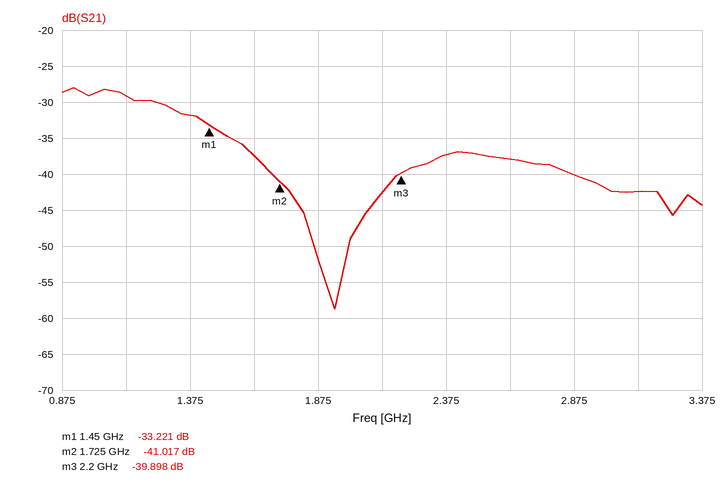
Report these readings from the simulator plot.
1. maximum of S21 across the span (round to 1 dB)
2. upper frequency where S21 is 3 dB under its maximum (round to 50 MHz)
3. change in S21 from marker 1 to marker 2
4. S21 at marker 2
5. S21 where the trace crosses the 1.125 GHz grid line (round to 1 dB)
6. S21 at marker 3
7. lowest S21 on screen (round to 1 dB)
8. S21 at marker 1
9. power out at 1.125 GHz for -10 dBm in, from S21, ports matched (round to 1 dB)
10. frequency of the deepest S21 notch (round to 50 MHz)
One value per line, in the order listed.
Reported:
-28 dB
1.30 GHz
-7.796 dB
-41.017 dB
-29 dB
-39.898 dB
-59 dB
-33.221 dB
-39 dBm
1.95 GHz
